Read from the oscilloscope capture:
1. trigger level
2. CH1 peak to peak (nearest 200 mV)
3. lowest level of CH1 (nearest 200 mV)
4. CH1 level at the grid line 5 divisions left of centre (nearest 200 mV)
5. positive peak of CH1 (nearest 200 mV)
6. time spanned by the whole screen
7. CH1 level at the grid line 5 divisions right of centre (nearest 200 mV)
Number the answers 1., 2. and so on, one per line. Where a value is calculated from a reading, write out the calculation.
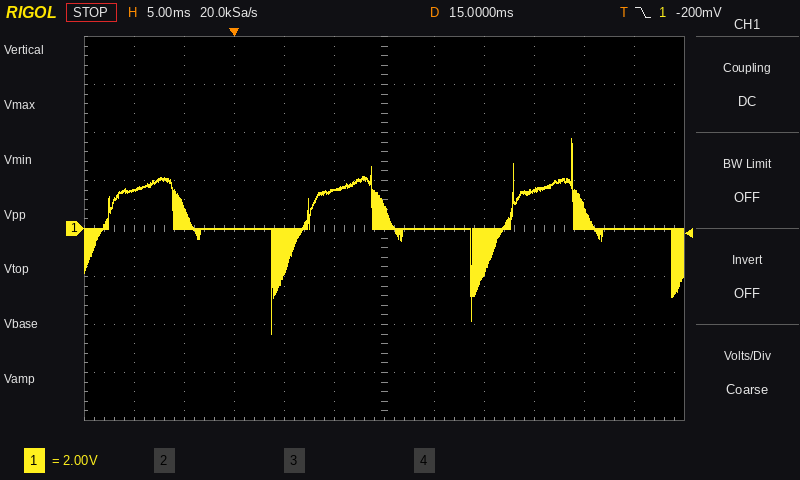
1. -200 mV
2. 3.8 V − (-4.4 V) = 8.2 V
3. -4.4 V
4. 1.6 V
5. 3.8 V
6. 60 ms
7. 0.0 V
